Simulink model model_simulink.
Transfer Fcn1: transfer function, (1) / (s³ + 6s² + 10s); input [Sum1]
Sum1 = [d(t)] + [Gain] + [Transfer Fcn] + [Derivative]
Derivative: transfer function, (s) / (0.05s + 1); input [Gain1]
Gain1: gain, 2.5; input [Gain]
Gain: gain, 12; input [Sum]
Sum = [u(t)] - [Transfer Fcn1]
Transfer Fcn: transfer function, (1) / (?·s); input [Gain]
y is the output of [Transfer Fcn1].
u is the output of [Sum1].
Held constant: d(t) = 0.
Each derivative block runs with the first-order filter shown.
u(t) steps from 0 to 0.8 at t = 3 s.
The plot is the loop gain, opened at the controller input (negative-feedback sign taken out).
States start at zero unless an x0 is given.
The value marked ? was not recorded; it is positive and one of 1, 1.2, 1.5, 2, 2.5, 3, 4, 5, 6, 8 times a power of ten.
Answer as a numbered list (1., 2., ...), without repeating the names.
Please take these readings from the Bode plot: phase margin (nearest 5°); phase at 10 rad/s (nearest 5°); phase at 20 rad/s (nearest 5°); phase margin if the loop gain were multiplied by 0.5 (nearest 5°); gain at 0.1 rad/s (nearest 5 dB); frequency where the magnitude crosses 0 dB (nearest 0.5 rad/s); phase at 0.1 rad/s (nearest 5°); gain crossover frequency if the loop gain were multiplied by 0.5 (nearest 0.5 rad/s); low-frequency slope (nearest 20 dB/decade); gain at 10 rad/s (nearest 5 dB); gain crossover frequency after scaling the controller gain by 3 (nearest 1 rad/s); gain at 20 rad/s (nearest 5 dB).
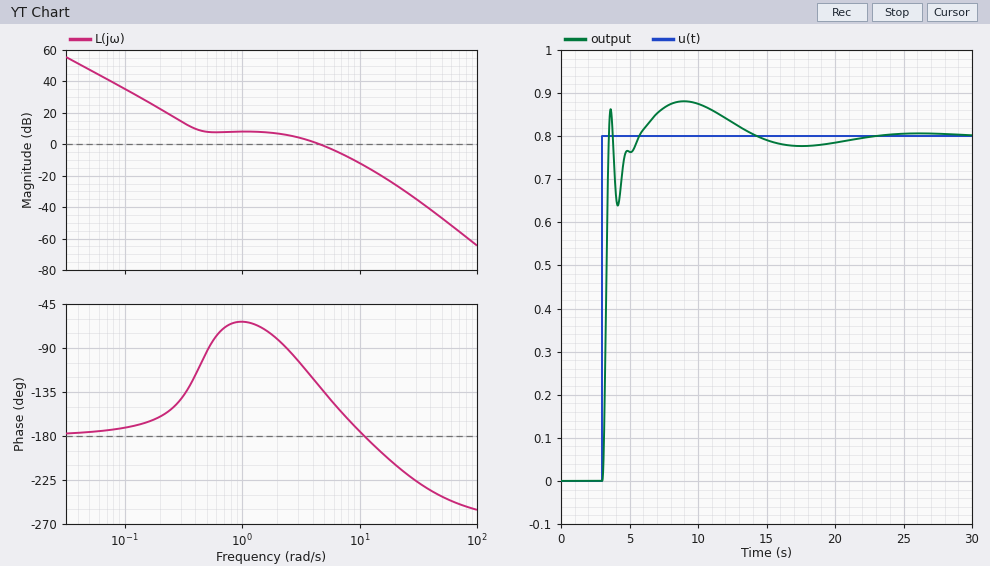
1. 50°
2. -175°
3. -210°
4. 90°
5. 35 dB
6. 4.5 rad/s
7. -170°
8. 2.5 rad/s
9. -40 dB/decade
10. -10 dB
11. 9 rad/s
12. -25 dB
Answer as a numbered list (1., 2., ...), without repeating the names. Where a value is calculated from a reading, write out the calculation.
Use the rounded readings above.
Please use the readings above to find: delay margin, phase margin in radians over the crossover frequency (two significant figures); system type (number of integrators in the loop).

1. 50 × π / 180 / 4.5 = 0.19 s
2. 2
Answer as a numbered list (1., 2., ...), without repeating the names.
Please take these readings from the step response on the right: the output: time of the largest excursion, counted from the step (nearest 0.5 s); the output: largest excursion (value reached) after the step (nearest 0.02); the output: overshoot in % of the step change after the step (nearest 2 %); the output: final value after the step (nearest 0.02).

1. 6.0 s
2. 0.88
3. 10 %
4. 0.80
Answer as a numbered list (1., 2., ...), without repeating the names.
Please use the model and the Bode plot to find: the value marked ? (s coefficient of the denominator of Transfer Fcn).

1. 2
